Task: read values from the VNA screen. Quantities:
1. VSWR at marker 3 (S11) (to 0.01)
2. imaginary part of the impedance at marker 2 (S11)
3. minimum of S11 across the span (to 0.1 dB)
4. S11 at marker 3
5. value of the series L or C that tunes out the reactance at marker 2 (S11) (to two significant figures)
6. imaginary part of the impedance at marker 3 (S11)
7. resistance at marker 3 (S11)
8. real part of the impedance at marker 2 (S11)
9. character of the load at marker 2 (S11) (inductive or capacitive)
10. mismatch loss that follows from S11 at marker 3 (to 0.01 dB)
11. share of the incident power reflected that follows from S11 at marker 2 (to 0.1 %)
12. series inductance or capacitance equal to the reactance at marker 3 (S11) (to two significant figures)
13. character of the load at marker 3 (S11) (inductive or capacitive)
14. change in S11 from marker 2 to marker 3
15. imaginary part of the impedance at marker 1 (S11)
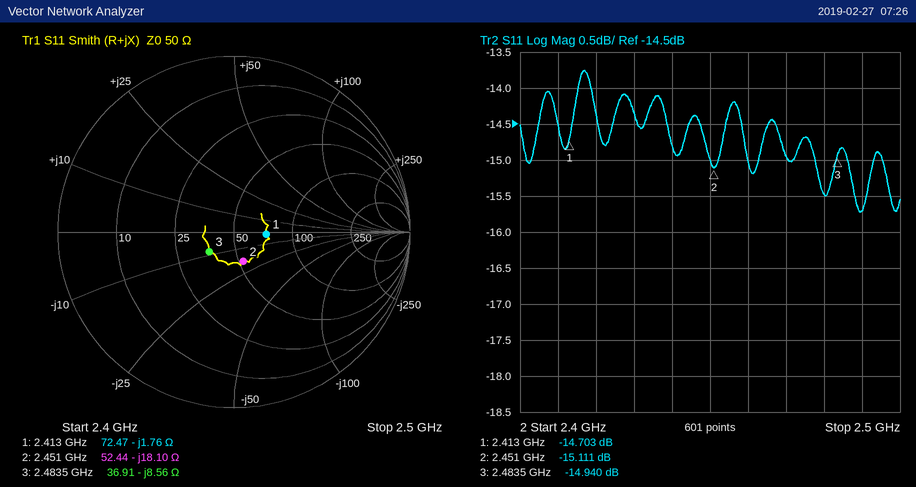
1.44
-18.10 Ω
-15.7 dB
-14.940 dB
1.2 nH
-8.56 Ω
36.91 Ω
52.44 Ω
capacitive
0.14 dB
3.1 %
7.5 pF
capacitive
0.171 dB
-1.76 Ω
